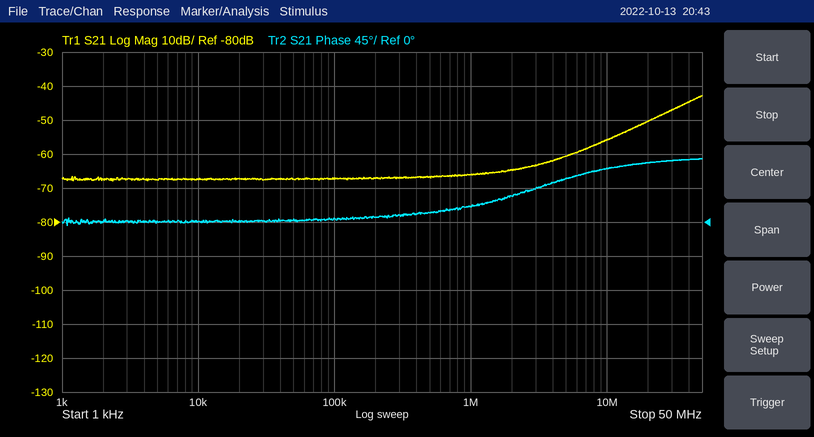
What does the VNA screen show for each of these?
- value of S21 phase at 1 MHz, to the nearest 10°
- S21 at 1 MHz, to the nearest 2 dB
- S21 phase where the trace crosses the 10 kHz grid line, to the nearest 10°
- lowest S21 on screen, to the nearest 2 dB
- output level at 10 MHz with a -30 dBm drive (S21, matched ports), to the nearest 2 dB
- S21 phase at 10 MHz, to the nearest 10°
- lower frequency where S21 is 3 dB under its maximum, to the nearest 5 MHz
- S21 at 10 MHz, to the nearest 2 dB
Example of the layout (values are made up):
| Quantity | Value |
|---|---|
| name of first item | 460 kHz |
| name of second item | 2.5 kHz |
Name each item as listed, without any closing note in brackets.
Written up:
| Quantity | Value |
|---|---|
| value of S21 phase at 1 MHz, to the nearest 10° | 20° |
| S21 at 1 MHz, to the nearest 2 dB | -66 dB |
| S21 phase where the trace crosses the 10 kHz grid line, to the nearest 10° | 0° |
| lowest S21 on screen, to the nearest 2 dB | -68 dB |
| output level at 10 MHz with a -30 dBm drive (S21, matched ports), to the nearest 2 dB | -86 dBm |
| S21 phase at 10 MHz, to the nearest 10° | 70° |
| lower frequency where S21 is 3 dB under its maximum, to the nearest 5 MHz | 35 MHz |
| S21 at 10 MHz, to the nearest 2 dB | -56 dB |
